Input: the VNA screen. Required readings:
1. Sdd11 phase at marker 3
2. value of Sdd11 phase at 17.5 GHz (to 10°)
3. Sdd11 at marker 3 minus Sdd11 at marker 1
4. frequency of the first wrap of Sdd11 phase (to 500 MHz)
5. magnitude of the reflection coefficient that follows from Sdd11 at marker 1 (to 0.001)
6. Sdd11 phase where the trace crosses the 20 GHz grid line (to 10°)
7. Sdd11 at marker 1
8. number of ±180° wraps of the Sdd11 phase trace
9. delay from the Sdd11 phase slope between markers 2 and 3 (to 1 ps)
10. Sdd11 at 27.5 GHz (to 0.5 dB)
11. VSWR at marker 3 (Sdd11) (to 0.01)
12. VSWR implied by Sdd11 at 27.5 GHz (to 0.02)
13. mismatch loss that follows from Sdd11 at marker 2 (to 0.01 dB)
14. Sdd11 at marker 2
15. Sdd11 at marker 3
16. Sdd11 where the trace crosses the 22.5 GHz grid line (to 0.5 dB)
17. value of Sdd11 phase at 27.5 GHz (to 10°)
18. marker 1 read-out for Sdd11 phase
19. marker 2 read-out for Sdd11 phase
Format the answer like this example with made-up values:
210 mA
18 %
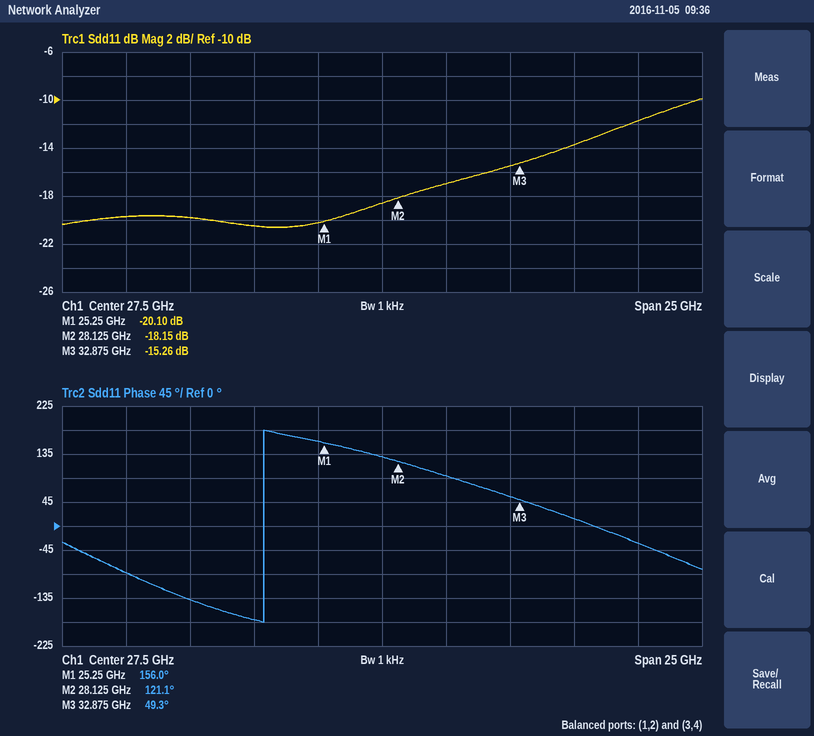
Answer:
49.3°
-90°
4.84 dB
23.0 GHz
0.099
-140°
-20.10 dB
1
42 ps
-18.5 dB
1.42
1.26
0.07 dB
-18.15 dB
-15.26 dB
-20.5 dB
130°
156.0°
121.1°
